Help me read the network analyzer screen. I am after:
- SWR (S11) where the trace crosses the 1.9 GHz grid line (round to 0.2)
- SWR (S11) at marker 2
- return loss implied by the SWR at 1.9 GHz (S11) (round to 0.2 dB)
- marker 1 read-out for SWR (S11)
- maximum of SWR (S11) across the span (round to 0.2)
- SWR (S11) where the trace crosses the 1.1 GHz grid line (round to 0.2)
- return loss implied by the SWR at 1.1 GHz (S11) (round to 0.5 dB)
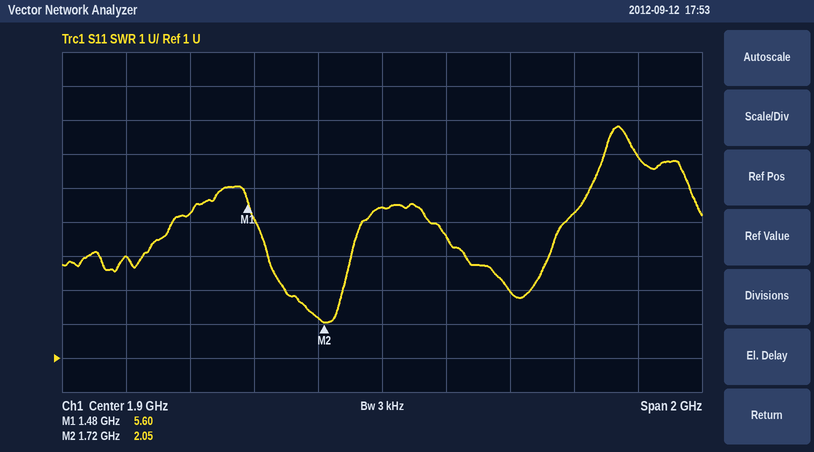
5.4
2.05
3.2 dB
5.60
7.8
4.0
4.5 dB
